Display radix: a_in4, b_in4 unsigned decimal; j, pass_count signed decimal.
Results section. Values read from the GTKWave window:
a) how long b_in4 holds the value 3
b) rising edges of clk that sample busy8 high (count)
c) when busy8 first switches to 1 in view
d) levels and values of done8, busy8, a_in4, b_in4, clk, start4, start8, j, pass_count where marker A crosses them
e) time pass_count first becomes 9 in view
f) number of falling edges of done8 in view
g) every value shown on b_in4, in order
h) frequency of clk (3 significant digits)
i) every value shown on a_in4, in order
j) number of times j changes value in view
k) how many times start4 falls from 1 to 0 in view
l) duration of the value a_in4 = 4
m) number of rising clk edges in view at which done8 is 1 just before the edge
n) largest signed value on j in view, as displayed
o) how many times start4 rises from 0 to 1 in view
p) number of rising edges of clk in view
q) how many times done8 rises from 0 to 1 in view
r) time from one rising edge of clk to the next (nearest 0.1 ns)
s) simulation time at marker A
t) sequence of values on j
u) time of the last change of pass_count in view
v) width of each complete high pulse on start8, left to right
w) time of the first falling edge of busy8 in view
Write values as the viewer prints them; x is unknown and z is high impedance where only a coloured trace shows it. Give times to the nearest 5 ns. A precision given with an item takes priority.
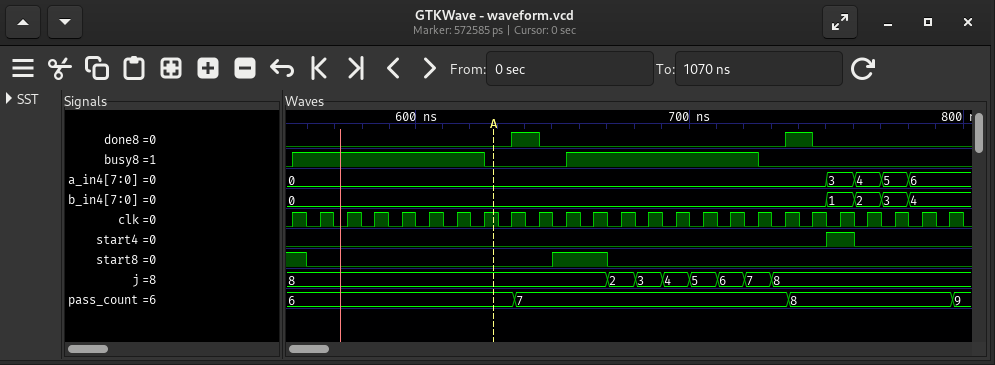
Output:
10 ns
14
555 ns
done8=0, busy8=0, a_in4=0, b_in4=0, clk=1, start4=0, start8=0, j=8, pass_count=6
795 ns
2
0, 1, 2, 3, 4
100 MHz
0, 3, 4, 5, 6
7
1
10 ns
2
8
1
25
2
10 ns
630 ns
8, 2, 3, 4, 5, 6, 7, 8
795 ns
20 ns
625 ns
